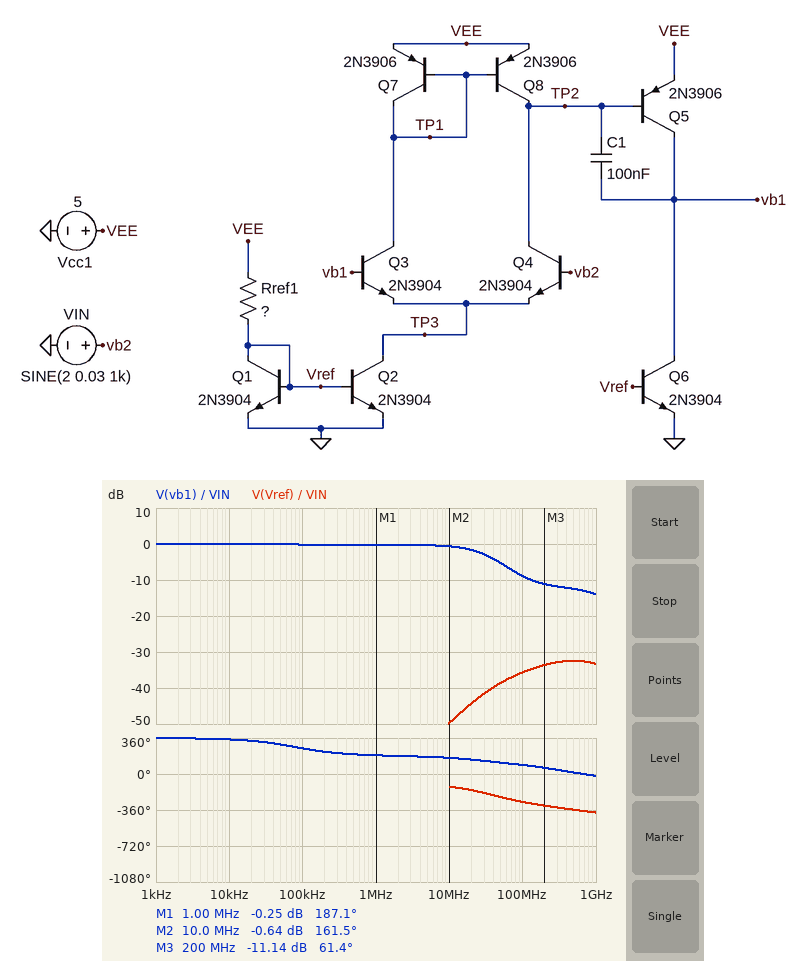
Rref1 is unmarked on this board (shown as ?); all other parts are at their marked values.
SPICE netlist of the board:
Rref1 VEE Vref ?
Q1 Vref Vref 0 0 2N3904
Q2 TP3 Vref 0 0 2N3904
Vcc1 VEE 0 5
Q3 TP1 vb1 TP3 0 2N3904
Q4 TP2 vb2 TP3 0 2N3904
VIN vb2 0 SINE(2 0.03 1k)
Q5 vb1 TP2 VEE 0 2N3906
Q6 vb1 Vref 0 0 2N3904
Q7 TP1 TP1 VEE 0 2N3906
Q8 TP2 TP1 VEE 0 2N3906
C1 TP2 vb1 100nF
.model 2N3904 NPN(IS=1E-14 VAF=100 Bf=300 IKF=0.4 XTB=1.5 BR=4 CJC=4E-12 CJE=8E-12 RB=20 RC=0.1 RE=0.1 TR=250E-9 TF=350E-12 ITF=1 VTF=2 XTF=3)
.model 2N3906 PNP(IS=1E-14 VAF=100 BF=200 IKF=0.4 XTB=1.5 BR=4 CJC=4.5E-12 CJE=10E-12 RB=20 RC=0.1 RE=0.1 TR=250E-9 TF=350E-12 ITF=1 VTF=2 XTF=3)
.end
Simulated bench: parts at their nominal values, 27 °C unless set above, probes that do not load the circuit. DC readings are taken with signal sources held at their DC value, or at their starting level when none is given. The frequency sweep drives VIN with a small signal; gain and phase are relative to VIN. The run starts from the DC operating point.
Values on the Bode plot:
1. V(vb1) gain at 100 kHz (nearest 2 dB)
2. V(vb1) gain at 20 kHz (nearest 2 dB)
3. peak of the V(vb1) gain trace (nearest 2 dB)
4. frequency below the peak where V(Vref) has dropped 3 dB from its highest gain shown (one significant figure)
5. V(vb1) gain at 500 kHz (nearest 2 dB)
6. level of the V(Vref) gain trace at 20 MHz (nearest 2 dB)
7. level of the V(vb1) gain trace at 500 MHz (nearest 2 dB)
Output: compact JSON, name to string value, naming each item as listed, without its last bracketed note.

{"V(vb1) gain at 100 kHz": "0 dB", "V(vb1) gain at 20 kHz": "0 dB", "peak of the V(vb1) gain trace": "0 dB", "frequency below the peak where V(Vref) has dropped 3 dB from its highest gain shown": "100 MHz", "V(vb1) gain at 500 kHz": "0 dB", "level of the V(Vref) gain trace at 20 MHz": "-44 dB", "level of the V(vb1) gain trace at 500 MHz": "-12 dB"}
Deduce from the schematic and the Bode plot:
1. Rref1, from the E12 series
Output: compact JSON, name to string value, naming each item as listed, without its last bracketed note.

{"Rref1, from the E12 series": "3.3 kΩ"}
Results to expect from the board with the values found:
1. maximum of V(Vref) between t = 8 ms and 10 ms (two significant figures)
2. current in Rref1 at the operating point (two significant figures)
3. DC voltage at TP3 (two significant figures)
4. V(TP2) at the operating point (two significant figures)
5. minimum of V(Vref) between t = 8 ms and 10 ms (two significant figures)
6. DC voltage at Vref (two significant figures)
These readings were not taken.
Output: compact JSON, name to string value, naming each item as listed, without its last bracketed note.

{"maximum of V(Vref) between t = 8 ms and 10 ms": "660 mV", "current in Rref1 at the operating point": "1.3 mA", "DC voltage at TP3": "1.4 V", "V(TP2) at the operating point": "4.3 V", "minimum of V(Vref) between t = 8 ms and 10 ms": "660 mV", "DC voltage at Vref": "660 mV"}
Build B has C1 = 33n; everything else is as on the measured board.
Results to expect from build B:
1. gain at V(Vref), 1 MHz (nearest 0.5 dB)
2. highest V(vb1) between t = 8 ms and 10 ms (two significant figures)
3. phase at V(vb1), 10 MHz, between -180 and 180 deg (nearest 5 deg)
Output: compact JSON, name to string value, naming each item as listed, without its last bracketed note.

{"gain at V(Vref), 1 MHz": "-68.5 dB", "highest V(vb1) between t = 8 ms and 10 ms": "2.0 V", "phase at V(vb1), 10 MHz, between -180 and 180 deg": "165 deg"}
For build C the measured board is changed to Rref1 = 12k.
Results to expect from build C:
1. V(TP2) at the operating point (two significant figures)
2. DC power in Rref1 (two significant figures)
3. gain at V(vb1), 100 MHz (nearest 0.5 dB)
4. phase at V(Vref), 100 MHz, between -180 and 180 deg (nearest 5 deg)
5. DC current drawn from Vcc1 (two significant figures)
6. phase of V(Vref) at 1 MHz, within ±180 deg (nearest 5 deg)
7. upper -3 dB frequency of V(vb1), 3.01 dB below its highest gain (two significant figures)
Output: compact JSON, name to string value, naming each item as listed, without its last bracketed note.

{"V(TP2) at the operating point": "4.4 V", "DC power in Rref1": "1.6 mW", "gain at V(vb1), 100 MHz": "-12.0 dB", "phase at V(Vref), 100 MHz, between -180 and 180 deg": "40 deg", "DC current drawn from Vcc1": "1.1 mA", "phase of V(Vref) at 1 MHz, within ±180 deg": "-95 deg", "upper -3 dB frequency of V(vb1), 3.01 dB below its highest gain": "11 MHz"}
